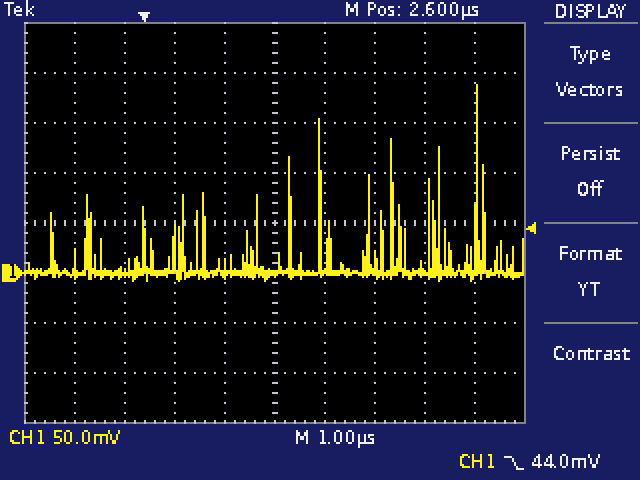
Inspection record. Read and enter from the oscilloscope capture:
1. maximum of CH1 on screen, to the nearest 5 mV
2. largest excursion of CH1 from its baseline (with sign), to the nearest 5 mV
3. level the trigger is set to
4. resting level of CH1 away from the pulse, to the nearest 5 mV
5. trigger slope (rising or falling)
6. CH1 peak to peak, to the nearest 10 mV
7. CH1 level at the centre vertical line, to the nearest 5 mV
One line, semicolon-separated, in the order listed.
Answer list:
190 mV; +190 mV; 44.0 mV; 0 mV; falling; 200 mV; 0 mV
